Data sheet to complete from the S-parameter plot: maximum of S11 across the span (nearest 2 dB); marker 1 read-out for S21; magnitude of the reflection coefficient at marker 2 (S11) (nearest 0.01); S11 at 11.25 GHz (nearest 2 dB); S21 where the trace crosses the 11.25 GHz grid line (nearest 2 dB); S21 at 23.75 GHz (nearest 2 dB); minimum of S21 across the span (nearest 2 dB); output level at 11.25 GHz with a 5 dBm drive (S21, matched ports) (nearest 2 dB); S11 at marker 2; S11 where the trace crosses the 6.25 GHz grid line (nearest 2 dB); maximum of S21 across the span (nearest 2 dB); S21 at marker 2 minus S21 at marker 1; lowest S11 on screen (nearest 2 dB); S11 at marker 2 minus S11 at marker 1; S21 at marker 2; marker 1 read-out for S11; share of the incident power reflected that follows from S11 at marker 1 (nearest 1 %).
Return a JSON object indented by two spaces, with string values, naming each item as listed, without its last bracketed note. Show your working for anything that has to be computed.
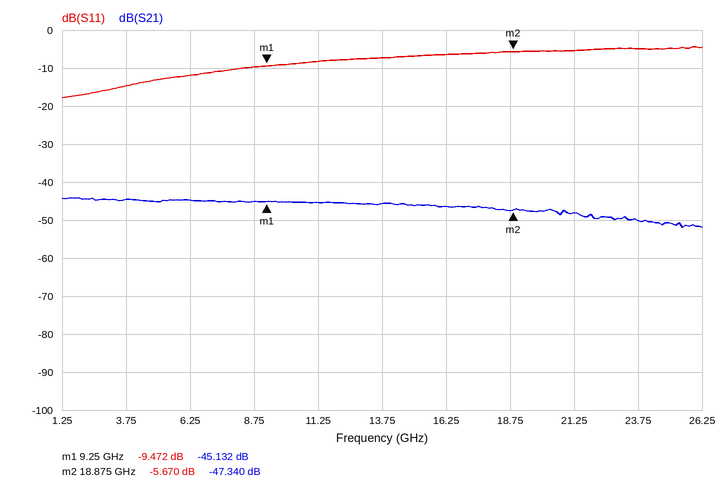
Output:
{
  "maximum of S11 across the span": "-4 dB",
  "marker 1 read-out for S21": "-45.132 dB",
  "magnitude of the reflection coefficient at marker 2 (S11)": "10^(-5.67/20) ≈ 0.52",
  "S11 at 11.25 GHz": "-8 dB",
  "S21 where the trace crosses the 11.25 GHz grid line": "-46 dB",
  "S21 at 23.75 GHz": "-50 dB",
  "minimum of S21 across the span": "-52 dB",
  "output level at 11.25 GHz with a 5 dBm drive (S21, matched ports)": "5 dBm + (-46 dB) = -40 dBm",
  "S11 at marker 2": "-5.670 dB",
  "S11 where the trace crosses the 6.25 GHz grid line": "-12 dB",
  "maximum of S21 across the span": "-44 dB",
  "S21 at marker 2 minus S21 at marker 1": "-47.34 − (-45.132) = -2.208 dB",
  "lowest S11 on screen": "-18 dB",
  "S11 at marker 2 minus S11 at marker 1": "-5.67 − (-9.472) = 3.802 dB",
  "S21 at marker 2": "-47.340 dB",
  "marker 1 read-out for S11": "-9.472 dB",
  "share of the incident power reflected that follows from S11 at marker 1": "10^(-9.472/10) ≈ 11 %"
}
